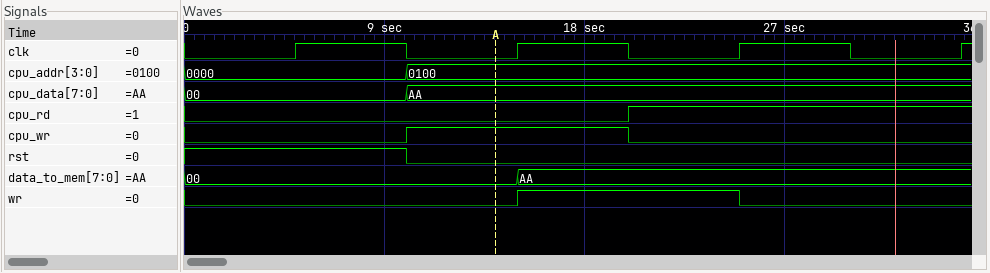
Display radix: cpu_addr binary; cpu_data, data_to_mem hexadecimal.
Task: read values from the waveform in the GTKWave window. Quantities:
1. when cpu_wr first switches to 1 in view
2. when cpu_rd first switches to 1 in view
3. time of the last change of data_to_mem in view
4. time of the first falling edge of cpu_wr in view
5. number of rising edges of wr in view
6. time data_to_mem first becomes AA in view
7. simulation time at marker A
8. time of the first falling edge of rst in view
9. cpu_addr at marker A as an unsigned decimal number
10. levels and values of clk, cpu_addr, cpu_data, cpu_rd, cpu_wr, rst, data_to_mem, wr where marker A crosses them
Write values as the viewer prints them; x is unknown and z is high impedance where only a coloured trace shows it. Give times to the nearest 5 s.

10 s
20 s
15 s
20 s
1
15 s
15 s
10 s
4
clk=0, cpu_addr=0100, cpu_data=AA, cpu_rd=0, cpu_wr=1, rst=0, data_to_mem=00, wr=0
